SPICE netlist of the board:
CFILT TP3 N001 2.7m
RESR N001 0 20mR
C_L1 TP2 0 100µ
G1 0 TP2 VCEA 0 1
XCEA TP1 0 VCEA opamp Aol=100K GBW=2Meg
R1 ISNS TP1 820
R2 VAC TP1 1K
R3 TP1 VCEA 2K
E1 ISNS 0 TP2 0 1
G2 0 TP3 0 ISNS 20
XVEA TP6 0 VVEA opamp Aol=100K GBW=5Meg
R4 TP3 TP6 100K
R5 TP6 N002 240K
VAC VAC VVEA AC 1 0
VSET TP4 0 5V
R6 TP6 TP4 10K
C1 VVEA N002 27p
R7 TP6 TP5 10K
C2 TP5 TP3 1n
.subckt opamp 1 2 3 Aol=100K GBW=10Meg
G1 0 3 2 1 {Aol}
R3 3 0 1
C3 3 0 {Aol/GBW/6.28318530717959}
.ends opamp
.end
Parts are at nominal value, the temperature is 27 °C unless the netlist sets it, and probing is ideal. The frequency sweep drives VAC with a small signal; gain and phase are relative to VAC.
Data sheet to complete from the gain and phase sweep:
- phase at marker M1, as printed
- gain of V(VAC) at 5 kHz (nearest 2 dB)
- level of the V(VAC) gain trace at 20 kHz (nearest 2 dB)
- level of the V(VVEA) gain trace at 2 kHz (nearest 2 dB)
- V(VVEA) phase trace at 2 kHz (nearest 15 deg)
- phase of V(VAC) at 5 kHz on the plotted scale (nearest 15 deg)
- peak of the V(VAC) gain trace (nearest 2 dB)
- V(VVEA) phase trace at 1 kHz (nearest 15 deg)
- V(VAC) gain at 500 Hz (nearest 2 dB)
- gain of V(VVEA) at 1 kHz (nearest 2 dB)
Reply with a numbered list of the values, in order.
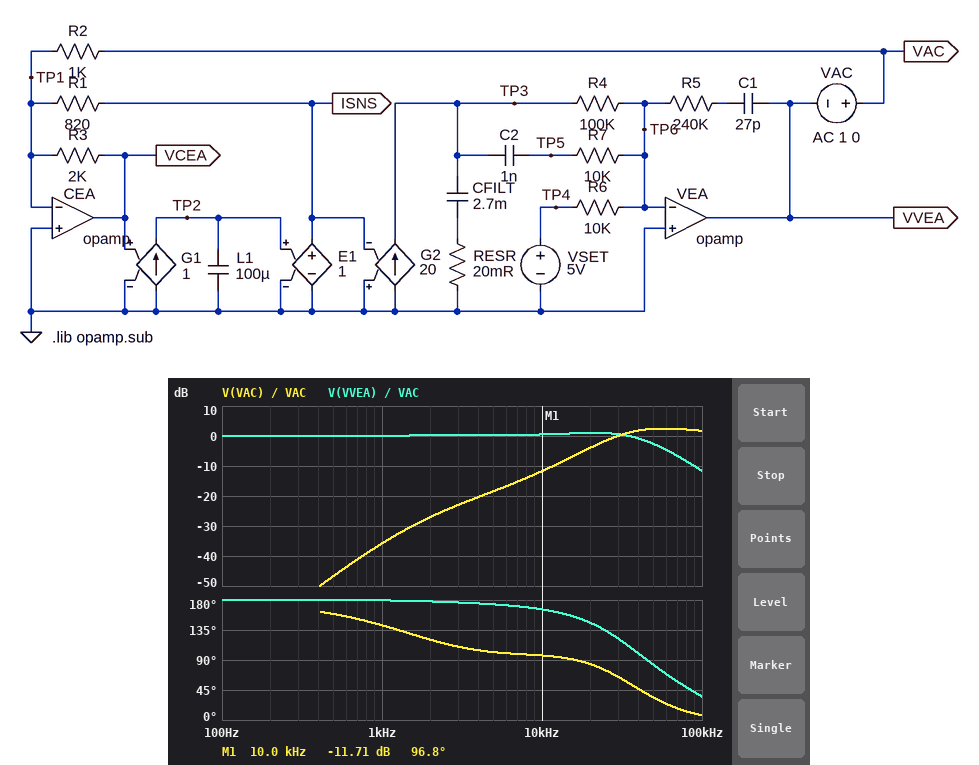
1. 96.8 deg
2. -18 dB
3. -4 dB
4. 0 dB
5. 180 deg
6. 105 deg
7. 2 dB
8. 180 deg
9. -46 dB
10. 0 dB
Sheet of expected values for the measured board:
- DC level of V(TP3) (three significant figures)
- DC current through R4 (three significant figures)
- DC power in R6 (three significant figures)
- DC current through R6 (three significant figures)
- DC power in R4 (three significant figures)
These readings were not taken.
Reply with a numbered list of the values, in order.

1. -50.0 V
2. 500 µA
3. 2.50 mW
4. 500 µA
5. 25.0 mW
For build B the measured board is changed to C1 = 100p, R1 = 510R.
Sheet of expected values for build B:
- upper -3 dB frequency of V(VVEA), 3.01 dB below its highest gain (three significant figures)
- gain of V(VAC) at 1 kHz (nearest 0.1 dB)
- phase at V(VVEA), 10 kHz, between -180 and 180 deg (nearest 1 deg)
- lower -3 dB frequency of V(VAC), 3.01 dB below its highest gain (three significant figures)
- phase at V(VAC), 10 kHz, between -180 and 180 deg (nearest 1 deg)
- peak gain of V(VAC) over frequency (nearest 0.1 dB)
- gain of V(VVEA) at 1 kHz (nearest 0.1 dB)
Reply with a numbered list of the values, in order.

1. 12.4 kHz
2. -21.0 dB
3. 159 deg
4. 38.0 kHz
5. 43 deg
6. 2.0 dB
7. 0.5 dB
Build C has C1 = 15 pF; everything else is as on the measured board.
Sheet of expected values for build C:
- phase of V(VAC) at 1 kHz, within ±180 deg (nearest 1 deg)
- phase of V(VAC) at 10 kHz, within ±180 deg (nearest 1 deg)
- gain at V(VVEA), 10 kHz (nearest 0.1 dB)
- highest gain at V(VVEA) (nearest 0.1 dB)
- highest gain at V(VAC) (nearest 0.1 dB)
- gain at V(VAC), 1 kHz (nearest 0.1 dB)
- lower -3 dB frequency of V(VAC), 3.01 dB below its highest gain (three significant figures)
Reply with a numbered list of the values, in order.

1. 143 deg
2. 113 deg
3. 0.7 dB
4. 3.6 dB
5. 4.3 dB
6. -40.2 dB
7. 29.6 kHz
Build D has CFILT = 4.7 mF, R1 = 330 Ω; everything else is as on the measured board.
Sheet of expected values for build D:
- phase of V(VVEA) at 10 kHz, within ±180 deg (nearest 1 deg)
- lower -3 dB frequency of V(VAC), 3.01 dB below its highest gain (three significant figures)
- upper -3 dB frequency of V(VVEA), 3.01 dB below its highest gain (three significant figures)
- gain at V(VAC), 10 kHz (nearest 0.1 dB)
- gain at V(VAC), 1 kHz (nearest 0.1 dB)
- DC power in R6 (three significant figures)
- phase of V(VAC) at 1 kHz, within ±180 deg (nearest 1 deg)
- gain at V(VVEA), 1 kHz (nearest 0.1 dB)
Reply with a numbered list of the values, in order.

1. 163 deg
2. 32.0 kHz
3. 48.3 kHz
4. -10.7 dB
5. -24.0 dB
6. 2.50 mW
7. 119 deg
8. 0.3 dB
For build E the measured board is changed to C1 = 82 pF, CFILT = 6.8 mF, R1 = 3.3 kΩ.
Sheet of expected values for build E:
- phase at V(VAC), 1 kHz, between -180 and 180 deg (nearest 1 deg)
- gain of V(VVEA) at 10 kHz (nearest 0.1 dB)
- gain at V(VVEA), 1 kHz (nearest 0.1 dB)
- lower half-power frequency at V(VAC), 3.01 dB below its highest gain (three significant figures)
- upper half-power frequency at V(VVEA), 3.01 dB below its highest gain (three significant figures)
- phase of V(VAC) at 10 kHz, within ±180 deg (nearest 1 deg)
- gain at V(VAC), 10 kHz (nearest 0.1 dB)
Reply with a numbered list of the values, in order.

1. 147 deg
2. -1.0 dB
3. 0.2 dB
4. 34.4 kHz
5. 33.3 kHz
6. 63 deg
7. -8.0 dB
